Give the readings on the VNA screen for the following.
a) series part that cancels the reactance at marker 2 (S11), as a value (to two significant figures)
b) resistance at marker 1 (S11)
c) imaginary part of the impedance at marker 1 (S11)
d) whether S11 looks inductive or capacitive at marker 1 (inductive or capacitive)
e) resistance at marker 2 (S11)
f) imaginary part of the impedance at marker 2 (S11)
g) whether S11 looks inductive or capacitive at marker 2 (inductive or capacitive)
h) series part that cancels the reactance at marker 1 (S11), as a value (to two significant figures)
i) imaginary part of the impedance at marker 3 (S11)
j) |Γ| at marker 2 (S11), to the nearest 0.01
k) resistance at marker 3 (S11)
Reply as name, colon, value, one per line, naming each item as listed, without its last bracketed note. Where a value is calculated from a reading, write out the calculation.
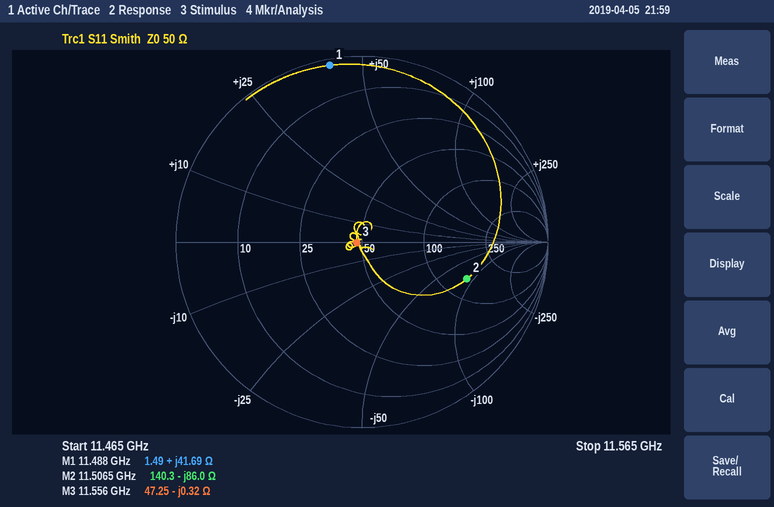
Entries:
series part that cancels the reactance at marker 2 (S11), as a value: L = 86 Ω/(2π × 11.5065 GHz) ≈ 1.2 nH
resistance at marker 1: 1.49 Ω
imaginary part of the impedance at marker 1: +41.69 Ω
whether S11 looks inductive or capacitive at marker 1: inductive
resistance at marker 2: 140.3 Ω
imaginary part of the impedance at marker 2: -86.0 Ω
whether S11 looks inductive or capacitive at marker 2: capacitive
series part that cancels the reactance at marker 1 (S11), as a value: C = 1/(2π × 11.488 GHz × 41.69 Ω) ≈ 332 fF, so 330 fF to two significant figures
imaginary part of the impedance at marker 3: -0.32 Ω
|Γ| at marker 2 (S11), to the nearest 0.01: 0.60
resistance at marker 3: 47.25 Ω
